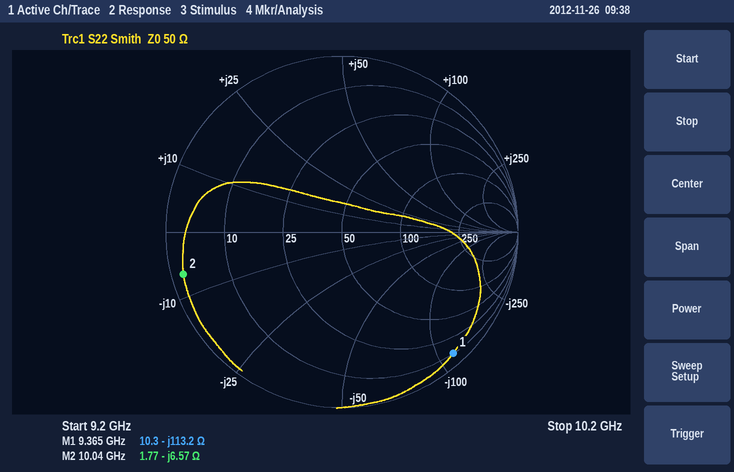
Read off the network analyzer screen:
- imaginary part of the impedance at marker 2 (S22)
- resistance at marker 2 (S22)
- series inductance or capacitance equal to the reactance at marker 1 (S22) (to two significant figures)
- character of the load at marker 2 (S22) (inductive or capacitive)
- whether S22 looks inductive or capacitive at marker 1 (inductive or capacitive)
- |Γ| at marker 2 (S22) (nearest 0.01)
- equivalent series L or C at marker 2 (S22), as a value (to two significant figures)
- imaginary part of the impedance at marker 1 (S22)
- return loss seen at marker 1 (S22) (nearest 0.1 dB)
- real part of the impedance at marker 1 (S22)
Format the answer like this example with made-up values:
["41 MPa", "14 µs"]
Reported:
["-6.57 Ω", "1.77 Ω", "150 fF", "capacitive", "capacitive", "0.93", "2.4 pF", "-113.2 Ω", "0.6 dB", "10.3 Ω"]
